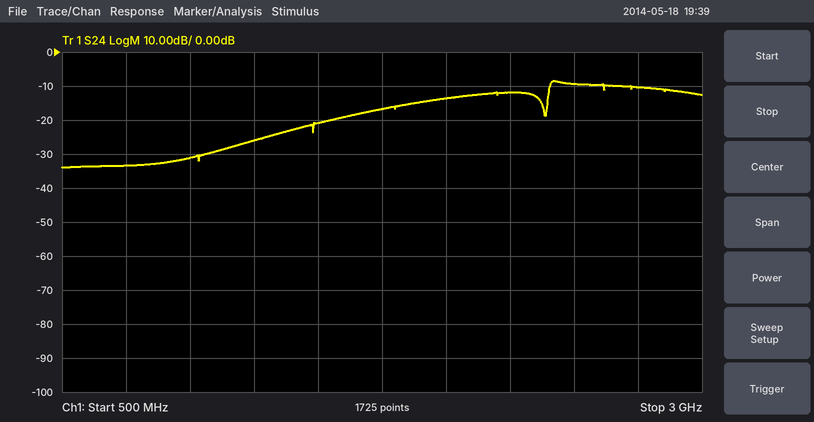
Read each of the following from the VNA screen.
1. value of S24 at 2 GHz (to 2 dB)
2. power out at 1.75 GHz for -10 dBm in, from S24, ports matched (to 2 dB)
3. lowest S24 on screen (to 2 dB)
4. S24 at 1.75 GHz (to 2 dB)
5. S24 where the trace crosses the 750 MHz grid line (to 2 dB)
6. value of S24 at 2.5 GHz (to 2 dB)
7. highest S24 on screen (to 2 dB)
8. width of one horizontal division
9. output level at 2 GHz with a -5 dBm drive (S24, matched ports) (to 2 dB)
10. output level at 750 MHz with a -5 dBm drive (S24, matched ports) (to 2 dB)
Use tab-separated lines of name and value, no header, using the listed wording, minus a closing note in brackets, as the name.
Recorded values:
value of S24 at 2 GHz	-14 dB
power out at 1.75 GHz for -10 dBm in, from S24, ports matched	-26 dBm
lowest S24 on screen	-34 dB
S24 at 1.75 GHz	-16 dB
S24 where the trace crosses the 750 MHz grid line	-34 dB
value of S24 at 2.5 GHz	-10 dB
highest S24 on screen	-8 dB
width of one horizontal division	250 MHz
output level at 2 GHz with a -5 dBm drive (S24, matched ports)	-18 dBm
output level at 750 MHz with a -5 dBm drive (S24, matched ports)	-38 dBm
